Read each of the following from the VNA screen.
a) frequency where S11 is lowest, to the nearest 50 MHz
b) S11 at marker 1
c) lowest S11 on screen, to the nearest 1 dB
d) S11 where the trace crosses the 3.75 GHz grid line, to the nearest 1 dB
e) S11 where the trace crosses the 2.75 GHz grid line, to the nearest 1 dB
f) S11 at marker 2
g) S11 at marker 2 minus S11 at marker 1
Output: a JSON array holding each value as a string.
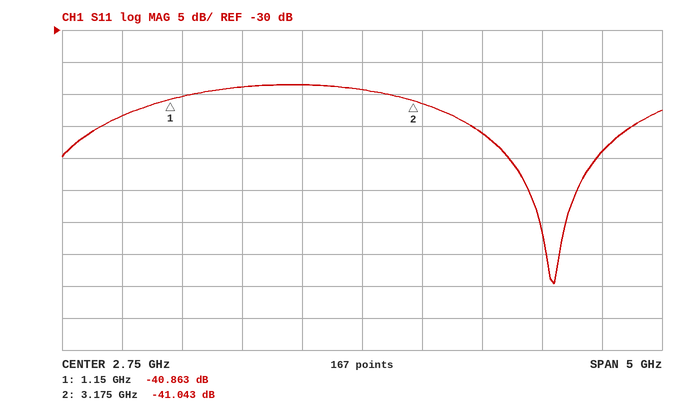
["4.35 GHz", "-40.863 dB", "-70 dB", "-46 dB", "-39 dB", "-41.043 dB", "-0.180 dB"]
